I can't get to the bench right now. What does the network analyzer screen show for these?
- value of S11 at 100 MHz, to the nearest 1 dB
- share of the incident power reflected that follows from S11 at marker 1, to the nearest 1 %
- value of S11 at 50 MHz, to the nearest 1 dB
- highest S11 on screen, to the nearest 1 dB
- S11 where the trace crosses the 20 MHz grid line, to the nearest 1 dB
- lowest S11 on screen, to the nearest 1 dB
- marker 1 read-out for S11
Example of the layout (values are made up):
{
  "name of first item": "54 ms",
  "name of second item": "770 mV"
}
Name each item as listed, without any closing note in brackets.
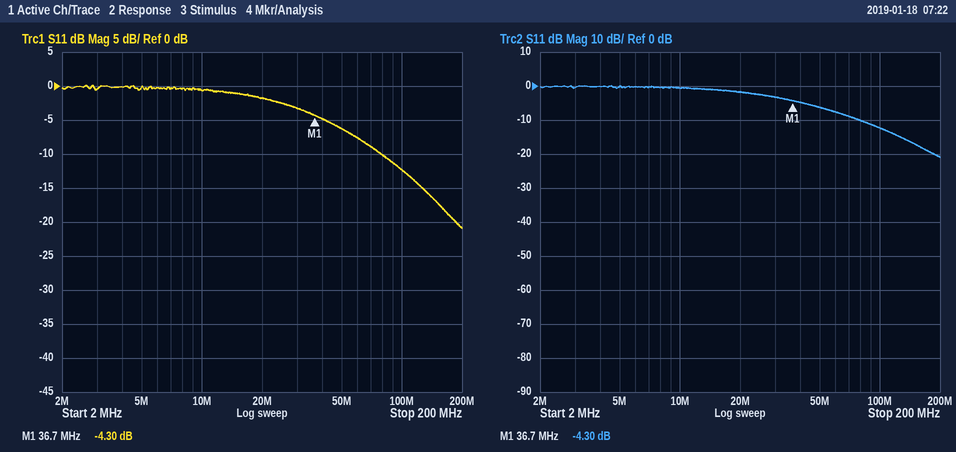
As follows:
{
  "value of S11 at 100 MHz, to the nearest 1 dB": "-12 dB",
  "share of the incident power reflected that follows from S11 at marker 1, to the nearest 1 %": "37 %",
  "value of S11 at 50 MHz, to the nearest 1 dB": "-6 dB",
  "highest S11 on screen, to the nearest 1 dB": "0 dB",
  "S11 where the trace crosses the 20 MHz grid line, to the nearest 1 dB": "-2 dB",
  "lowest S11 on screen, to the nearest 1 dB": "-21 dB",
  "marker 1 read-out for S11": "-4.30 dB"
}
